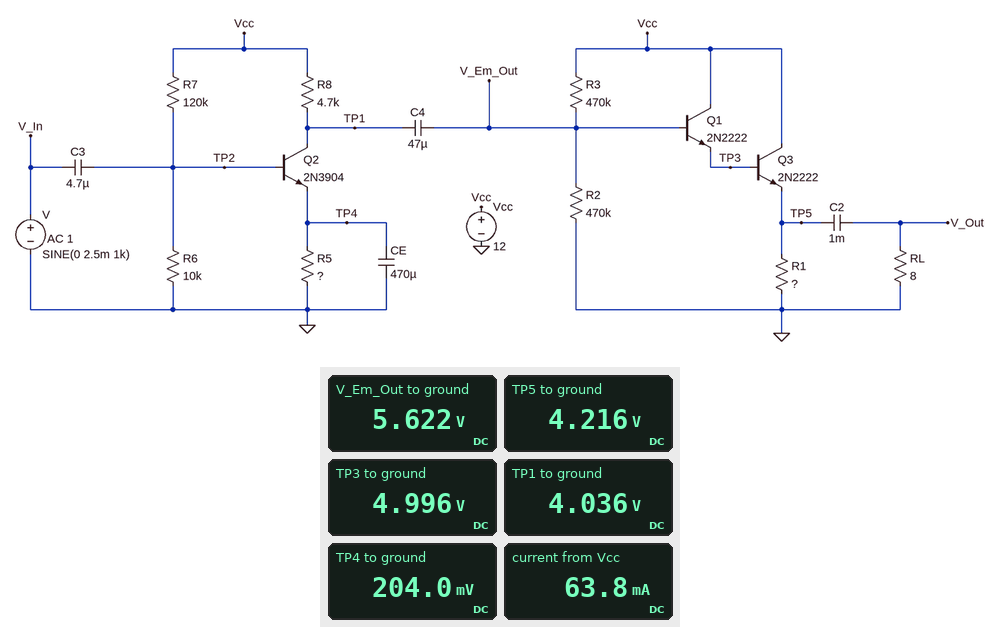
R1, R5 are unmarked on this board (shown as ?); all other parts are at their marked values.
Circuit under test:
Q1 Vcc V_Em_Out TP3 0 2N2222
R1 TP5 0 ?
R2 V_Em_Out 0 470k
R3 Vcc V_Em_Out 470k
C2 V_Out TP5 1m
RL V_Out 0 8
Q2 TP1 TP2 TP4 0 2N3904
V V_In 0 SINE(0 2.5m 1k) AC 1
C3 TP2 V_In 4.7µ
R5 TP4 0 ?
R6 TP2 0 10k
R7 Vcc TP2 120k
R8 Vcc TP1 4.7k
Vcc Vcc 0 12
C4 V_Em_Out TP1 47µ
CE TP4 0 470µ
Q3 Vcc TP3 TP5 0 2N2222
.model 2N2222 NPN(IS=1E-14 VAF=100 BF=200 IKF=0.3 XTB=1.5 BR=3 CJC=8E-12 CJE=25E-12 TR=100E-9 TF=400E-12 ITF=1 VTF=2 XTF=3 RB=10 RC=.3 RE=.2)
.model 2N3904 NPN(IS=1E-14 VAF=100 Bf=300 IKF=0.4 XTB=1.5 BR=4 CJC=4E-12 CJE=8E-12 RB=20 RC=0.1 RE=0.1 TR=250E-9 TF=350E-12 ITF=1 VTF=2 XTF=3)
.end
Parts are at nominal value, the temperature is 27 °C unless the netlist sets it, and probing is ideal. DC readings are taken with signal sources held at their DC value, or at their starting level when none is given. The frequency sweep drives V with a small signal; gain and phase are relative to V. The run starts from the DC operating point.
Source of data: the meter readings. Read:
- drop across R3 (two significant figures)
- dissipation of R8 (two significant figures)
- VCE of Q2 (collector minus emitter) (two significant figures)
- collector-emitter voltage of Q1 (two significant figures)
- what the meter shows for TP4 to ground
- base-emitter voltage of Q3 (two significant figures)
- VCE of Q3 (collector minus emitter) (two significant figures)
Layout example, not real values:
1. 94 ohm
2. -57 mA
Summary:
1. 6.4 V
2. 13 mW
3. 3.8 V
4. 7.0 V
5. 204.0 mV
6. 780 mV
7. 7.8 V
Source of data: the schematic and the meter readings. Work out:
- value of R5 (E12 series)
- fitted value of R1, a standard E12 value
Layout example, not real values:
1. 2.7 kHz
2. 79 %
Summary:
1. 120 Ω
2. 68 Ω
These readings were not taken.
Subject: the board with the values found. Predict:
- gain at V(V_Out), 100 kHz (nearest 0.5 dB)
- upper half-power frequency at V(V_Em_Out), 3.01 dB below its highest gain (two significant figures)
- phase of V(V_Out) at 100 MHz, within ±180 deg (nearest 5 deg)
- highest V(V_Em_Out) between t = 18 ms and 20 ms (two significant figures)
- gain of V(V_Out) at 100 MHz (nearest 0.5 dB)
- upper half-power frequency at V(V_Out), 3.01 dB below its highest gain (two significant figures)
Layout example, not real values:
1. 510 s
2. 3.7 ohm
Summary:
1. 47.5 dB
2. 3.8 MHz
3. 55 deg
4. 6.3 V
5. 1.5 dB
6. 3.7 MHz
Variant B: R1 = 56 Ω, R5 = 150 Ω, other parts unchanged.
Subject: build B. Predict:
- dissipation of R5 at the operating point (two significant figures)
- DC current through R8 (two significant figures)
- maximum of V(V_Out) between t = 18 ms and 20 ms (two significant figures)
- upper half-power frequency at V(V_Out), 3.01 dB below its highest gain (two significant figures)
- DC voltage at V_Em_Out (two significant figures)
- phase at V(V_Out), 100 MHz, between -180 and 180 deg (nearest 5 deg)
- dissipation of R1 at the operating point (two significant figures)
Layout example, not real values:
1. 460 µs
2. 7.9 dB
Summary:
1. 310 µW
2. 1.4 mA
3. 490 mV
4. 4.1 MHz
5. 5.5 V
6. 50 deg
7. 300 mW
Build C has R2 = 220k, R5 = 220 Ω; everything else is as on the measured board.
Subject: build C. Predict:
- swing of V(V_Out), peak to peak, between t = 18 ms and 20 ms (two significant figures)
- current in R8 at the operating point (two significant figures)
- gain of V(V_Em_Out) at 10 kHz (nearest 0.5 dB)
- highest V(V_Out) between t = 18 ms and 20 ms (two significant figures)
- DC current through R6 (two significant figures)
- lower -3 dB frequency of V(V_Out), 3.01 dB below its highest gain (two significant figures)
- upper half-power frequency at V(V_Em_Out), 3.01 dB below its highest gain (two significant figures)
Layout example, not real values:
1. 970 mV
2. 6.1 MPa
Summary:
1. 580 mV
2. 1.1 mA
3. 45.0 dB
4. 330 mV
5. 89 µA
6. 28 Hz
7. 3.9 MHz
